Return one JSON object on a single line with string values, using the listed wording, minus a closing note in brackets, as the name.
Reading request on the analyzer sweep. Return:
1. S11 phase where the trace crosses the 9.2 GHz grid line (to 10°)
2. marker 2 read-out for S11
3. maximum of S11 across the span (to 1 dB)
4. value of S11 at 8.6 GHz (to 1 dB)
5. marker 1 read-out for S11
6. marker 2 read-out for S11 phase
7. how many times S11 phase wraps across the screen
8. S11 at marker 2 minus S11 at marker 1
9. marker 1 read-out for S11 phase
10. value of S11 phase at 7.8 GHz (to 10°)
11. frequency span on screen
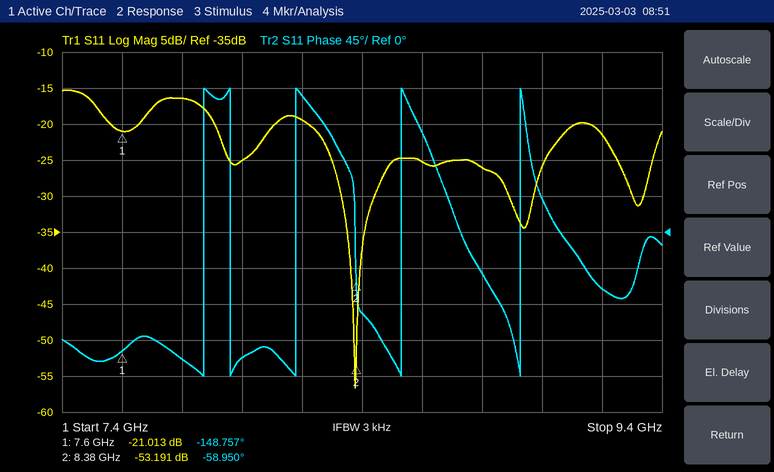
{"S11 phase where the trace crosses the 9.2 GHz grid line": "-70°", "marker 2 read-out for S11": "-53.191 dB", "maximum of S11 across the span": "-15 dB", "value of S11 at 8.6 GHz": "-25 dB", "marker 1 read-out for S11": "-21.013 dB", "marker 2 read-out for S11 phase": "-58.950°", "how many times S11 phase wraps across the screen": "5", "S11 at marker 2 minus S11 at marker 1": "-32.178 dB", "marker 1 read-out for S11 phase": "-148.757°", "value of S11 phase at 7.8 GHz": "-160°", "frequency span on screen": "2 GHz"}
